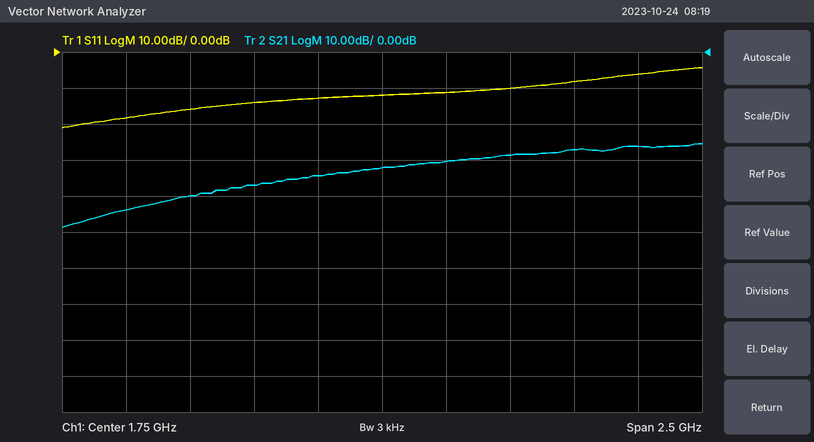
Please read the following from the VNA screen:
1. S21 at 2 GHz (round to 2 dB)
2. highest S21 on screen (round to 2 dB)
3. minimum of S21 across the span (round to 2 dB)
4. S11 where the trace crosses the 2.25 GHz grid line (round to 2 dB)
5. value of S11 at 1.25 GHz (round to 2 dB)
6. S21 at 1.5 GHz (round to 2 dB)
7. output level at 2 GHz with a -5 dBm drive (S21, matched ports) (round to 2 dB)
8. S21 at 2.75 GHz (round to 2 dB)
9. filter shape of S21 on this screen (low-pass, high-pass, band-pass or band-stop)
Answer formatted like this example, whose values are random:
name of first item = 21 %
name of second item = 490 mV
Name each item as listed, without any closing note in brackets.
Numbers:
S21 at 2 GHz = -30 dB
highest S21 on screen = -26 dB
minimum of S21 across the span = -48 dB
S11 where the trace crosses the 2.25 GHz grid line = -10 dB
value of S11 at 1.25 GHz = -14 dB
S21 at 1.5 GHz = -34 dB
output level at 2 GHz with a -5 dBm drive (S21, matched ports) = -36 dBm
S21 at 2.75 GHz = -26 dB
filter shape of S21 on this screen = high-pass
